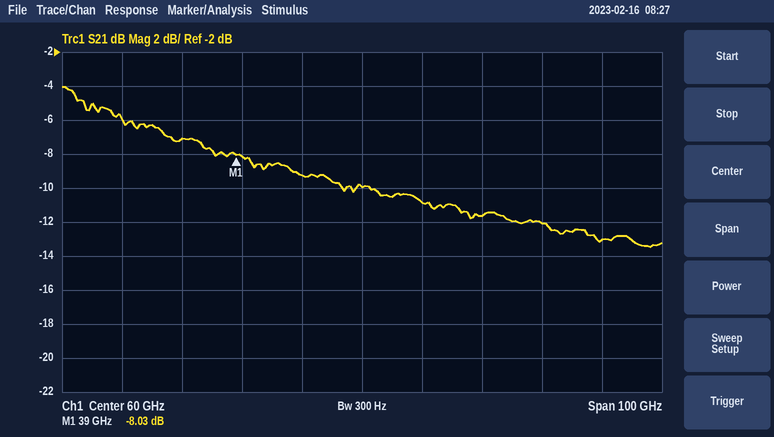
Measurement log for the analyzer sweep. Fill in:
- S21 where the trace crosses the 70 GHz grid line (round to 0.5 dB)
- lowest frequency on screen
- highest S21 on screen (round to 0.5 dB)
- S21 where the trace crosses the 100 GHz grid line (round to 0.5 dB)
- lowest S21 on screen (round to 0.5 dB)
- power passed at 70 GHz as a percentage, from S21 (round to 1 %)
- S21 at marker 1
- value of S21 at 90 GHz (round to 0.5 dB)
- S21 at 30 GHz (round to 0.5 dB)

-11.0 dB
10 GHz
-4.0 dB
-13.0 dB
-13.5 dB
8 %
-8.03 dB
-12.0 dB
-7.0 dB
